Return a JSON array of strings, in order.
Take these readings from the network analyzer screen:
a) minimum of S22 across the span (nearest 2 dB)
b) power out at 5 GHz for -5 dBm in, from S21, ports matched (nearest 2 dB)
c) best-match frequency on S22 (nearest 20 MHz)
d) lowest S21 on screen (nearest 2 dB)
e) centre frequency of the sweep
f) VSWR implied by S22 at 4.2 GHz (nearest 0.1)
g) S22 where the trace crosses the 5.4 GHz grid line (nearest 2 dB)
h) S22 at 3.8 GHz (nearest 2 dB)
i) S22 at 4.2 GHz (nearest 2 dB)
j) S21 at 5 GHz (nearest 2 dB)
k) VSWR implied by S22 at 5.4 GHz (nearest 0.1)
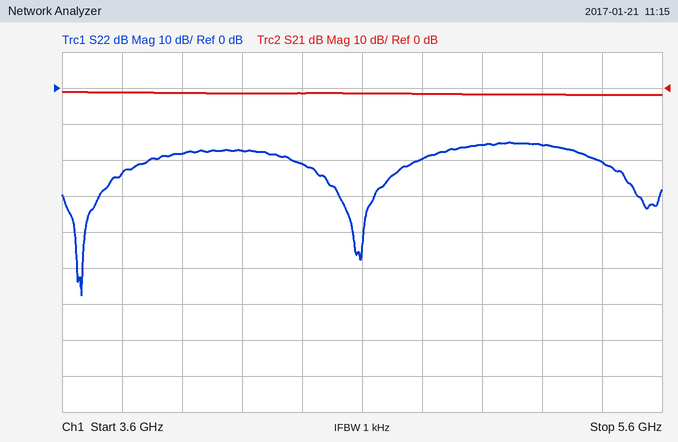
["-58 dB", "-6 dBm", "3.66 GHz", "-2 dB", "4.6 GHz", "1.3", "-20 dB", "-24 dB", "-18 dB", "-2 dB", "1.2"]
